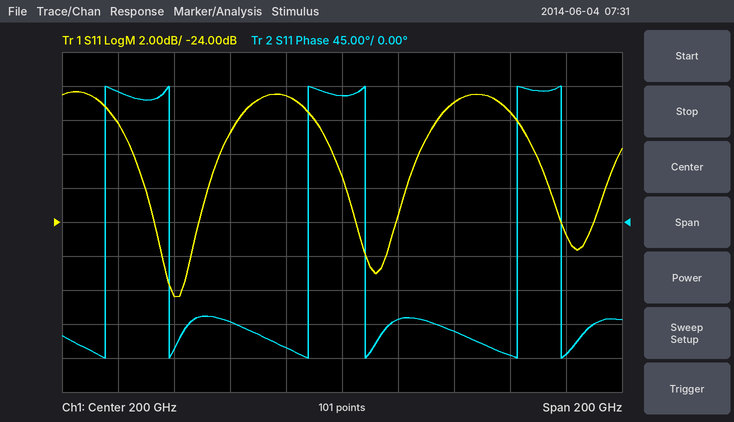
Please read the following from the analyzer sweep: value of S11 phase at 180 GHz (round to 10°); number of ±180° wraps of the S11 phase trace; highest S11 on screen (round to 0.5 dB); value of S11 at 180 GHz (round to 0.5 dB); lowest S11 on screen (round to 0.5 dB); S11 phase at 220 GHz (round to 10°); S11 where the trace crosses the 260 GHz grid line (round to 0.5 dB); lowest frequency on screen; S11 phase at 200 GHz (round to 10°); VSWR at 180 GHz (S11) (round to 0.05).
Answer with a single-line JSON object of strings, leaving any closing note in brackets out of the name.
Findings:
{"value of S11 phase at 180 GHz": "-170°", "number of ±180° wraps of the S11 phase trace": "6", "highest S11 on screen": "-16.5 dB", "value of S11 at 180 GHz": "-16.5 dB", "lowest S11 on screen": "-28.5 dB", "S11 phase at 220 GHz": "-130°", "S11 where the trace crosses the 260 GHz grid line": "-17.5 dB", "lowest frequency on screen": "100 GHz", "S11 phase at 200 GHz": "170°", "VSWR at 180 GHz (S11)": "1.35"}
